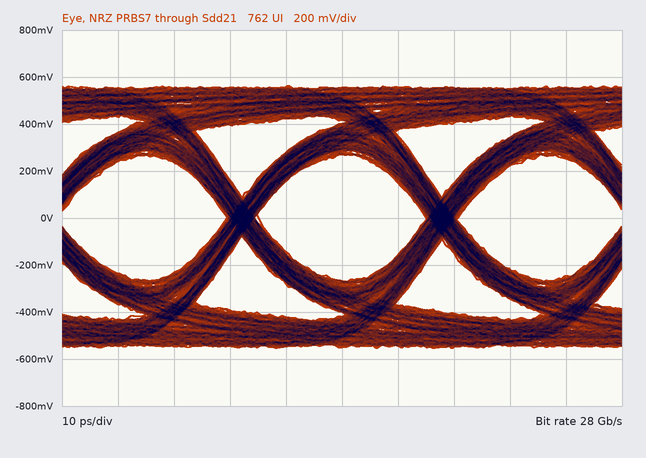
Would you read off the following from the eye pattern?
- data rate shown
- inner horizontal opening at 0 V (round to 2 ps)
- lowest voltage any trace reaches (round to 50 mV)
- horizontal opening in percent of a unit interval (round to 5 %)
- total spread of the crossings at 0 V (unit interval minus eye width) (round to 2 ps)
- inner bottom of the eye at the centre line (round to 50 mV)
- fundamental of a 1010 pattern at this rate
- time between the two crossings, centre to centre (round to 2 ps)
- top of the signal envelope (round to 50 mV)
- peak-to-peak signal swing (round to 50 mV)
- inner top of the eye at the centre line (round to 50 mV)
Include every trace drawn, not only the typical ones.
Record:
28 Gb/s
30 ps
-550 mV
85 %
6 ps
-250 mV
14 GHz
36 ps
550 mV
1.10 V
250 mV
